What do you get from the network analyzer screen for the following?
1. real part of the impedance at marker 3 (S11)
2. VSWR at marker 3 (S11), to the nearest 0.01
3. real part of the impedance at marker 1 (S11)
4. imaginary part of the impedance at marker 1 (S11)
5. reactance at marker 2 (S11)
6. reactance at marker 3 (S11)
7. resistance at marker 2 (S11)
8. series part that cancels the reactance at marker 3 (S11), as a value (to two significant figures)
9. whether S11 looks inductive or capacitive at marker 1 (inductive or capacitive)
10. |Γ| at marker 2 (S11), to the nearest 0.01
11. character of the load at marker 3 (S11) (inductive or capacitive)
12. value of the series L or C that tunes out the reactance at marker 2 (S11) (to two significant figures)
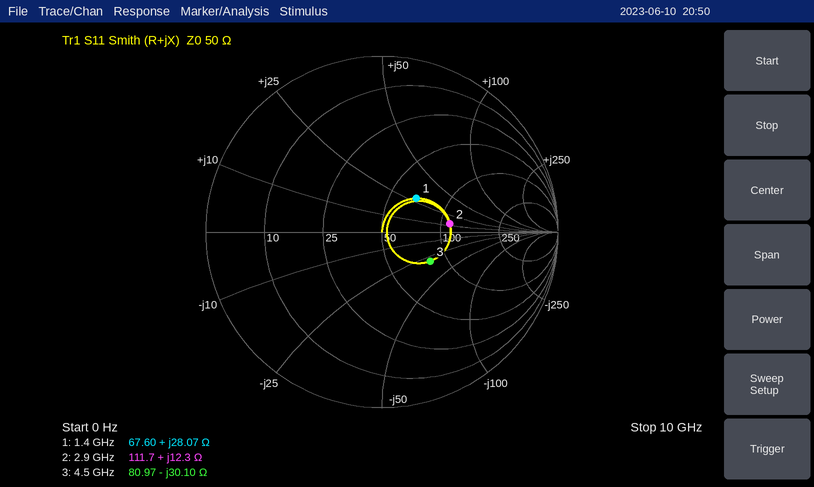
80.97 Ω
1.95
67.60 Ω
+28.07 Ω
+12.3 Ω
-30.10 Ω
111.7 Ω
1.1 nH
inductive
0.39
capacitive
4.5 pF
